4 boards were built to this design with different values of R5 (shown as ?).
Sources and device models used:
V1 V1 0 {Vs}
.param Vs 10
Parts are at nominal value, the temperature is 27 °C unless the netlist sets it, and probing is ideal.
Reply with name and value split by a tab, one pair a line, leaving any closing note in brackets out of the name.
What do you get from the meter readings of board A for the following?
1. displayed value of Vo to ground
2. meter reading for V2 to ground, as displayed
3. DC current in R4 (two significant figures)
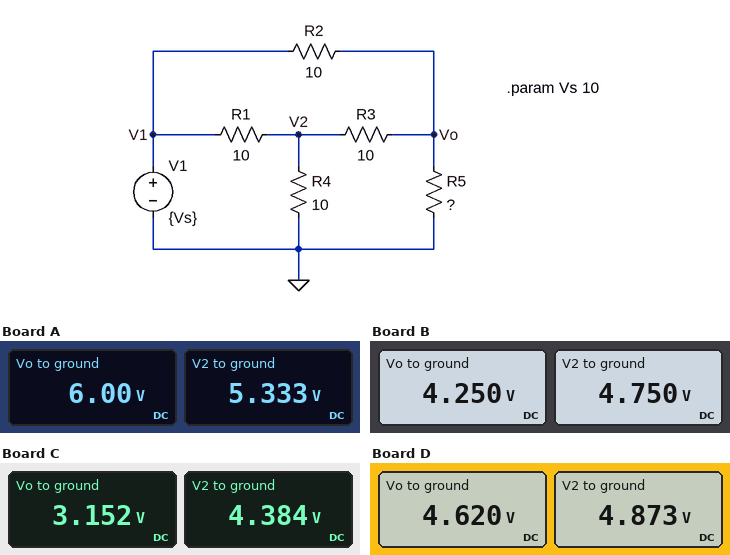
displayed value of Vo to ground	6.00 V
meter reading for V2 to ground, as displayed	5.333 V
DC current in R4	530 mA
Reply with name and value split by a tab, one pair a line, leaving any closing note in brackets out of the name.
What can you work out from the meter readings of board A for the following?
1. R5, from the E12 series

R5, from the E12 series	18 Ω
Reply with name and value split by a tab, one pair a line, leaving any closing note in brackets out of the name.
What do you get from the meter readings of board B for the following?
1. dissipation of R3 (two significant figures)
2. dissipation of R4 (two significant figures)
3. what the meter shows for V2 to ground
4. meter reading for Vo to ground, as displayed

dissipation of R3	25 mW
dissipation of R4	2.3 W
what the meter shows for V2 to ground	4.750 V
meter reading for Vo to ground, as displayed	4.250 V
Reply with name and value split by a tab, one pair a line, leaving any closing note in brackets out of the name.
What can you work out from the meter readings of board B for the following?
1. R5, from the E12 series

R5, from the E12 series	6.8 Ω
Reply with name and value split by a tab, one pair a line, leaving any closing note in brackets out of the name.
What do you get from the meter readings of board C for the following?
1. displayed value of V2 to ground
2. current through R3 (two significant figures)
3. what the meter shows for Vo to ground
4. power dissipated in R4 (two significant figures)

displayed value of V2 to ground	4.384 V
current through R3	120 mA
what the meter shows for Vo to ground	3.152 V
power dissipated in R4	1.9 W
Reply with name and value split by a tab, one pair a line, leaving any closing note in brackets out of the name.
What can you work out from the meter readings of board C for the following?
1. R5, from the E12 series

R5, from the E12 series	3.9 Ω
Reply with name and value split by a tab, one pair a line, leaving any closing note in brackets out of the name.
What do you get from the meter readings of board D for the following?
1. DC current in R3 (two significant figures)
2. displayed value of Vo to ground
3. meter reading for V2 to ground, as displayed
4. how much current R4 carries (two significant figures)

DC current in R3	25 mA
displayed value of Vo to ground	4.620 V
meter reading for V2 to ground, as displayed	4.873 V
how much current R4 carries	490 mA
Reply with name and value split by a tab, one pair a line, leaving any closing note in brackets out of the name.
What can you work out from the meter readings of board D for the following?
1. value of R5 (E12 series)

value of R5	8.2 Ω
